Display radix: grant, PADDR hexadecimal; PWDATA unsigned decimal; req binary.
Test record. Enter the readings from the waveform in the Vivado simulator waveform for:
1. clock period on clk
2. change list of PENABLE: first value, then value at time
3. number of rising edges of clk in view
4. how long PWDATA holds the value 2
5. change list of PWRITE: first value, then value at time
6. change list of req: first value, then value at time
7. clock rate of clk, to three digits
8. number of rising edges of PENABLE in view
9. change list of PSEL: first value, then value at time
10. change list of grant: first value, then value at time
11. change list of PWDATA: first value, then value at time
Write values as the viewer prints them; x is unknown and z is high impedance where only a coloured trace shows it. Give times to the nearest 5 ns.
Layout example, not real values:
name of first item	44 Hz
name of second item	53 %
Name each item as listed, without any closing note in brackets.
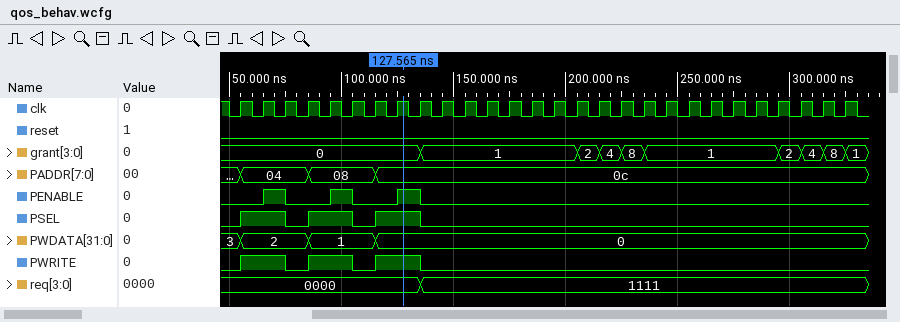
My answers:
clock period on clk	10 ns
change list of PENABLE: first value, then value at time	0, 1 at 65 ns, 0 at 75 ns, 1 at 95 ns, 0 at 105 ns, 1 at 125 ns, 0 at 135 ns
number of rising edges of clk in view	28
how long PWDATA holds the value 2	30 ns
change list of PWRITE: first value, then value at time	0, 1 at 55 ns, 0 at 75 ns, 1 at 85 ns, 0 at 105 ns, 1 at 115 ns, 0 at 135 ns
change list of req: first value, then value at time	0000, 1111 at 135 ns
clock rate of clk, to three digits	100 MHz
number of rising edges of PENABLE in view	3
change list of PSEL: first value, then value at time	0, 1 at 55 ns, 0 at 75 ns, 1 at 85 ns, 0 at 105 ns, 1 at 115 ns, 0 at 135 ns
change list of grant: first value, then value at time	0, 1 at 135 ns, 2 at 205 ns, 4 at 215 ns, 8 at 225 ns, 1 at 235 ns, 2 at 295 ns, 4 at 305 ns, 8 at 315 ns, 1 at 325 ns
change list of PWDATA: first value, then value at time	3, 2 at 55 ns, 1 at 85 ns, 0 at 115 ns
